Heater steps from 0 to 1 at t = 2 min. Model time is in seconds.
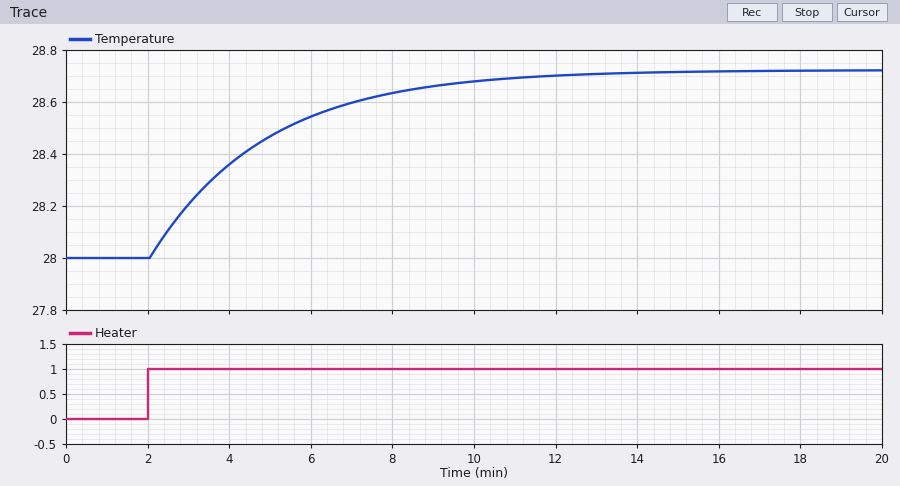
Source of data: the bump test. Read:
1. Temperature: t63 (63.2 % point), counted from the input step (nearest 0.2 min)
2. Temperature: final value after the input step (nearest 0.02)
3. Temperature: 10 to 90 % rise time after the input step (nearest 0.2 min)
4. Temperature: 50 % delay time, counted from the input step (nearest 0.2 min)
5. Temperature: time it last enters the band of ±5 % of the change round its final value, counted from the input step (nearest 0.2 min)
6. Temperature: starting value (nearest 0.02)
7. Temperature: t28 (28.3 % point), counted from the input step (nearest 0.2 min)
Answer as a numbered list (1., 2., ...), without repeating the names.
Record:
1. 2.8 min
2. 28.72
3. 6.2 min
4. 2.0 min
5. 8.6 min
6. 28.00
7. 1.0 min
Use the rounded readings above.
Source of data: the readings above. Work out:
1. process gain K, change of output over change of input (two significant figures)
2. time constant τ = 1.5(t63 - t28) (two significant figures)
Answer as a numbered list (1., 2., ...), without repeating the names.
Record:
1. 0.72
2. 2.7 min
